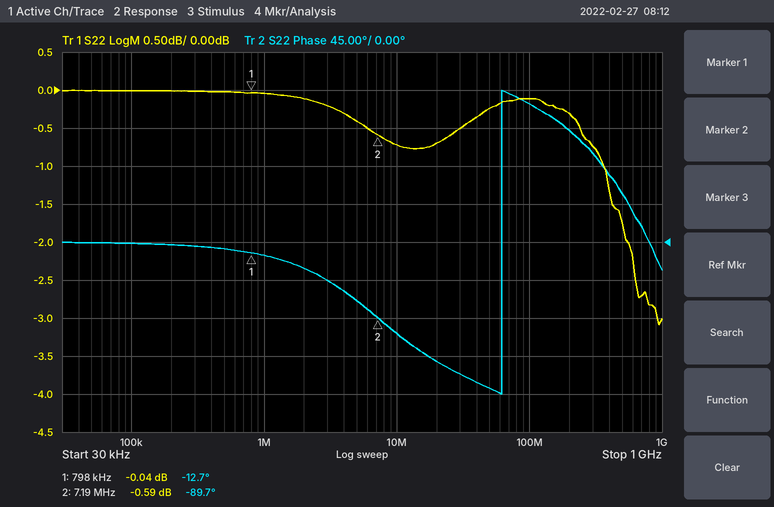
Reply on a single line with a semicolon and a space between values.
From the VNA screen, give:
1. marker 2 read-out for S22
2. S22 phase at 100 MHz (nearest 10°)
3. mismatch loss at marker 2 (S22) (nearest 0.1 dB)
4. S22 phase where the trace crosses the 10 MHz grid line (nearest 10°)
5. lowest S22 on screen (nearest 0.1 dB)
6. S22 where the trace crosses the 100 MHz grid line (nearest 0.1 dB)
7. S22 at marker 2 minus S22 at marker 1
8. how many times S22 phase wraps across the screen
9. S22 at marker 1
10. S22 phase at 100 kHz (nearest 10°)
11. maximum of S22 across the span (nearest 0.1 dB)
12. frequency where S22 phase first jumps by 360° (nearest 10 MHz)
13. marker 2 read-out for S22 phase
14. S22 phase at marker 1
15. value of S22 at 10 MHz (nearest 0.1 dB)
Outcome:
-0.59 dB; 160°; 9.0 dB; -110°; -3.1 dB; -0.1 dB; -0.55 dB; 1; -0.04 dB; 0°; 0.0 dB; 60 MHz; -89.7°; -12.7°; -0.7 dB
